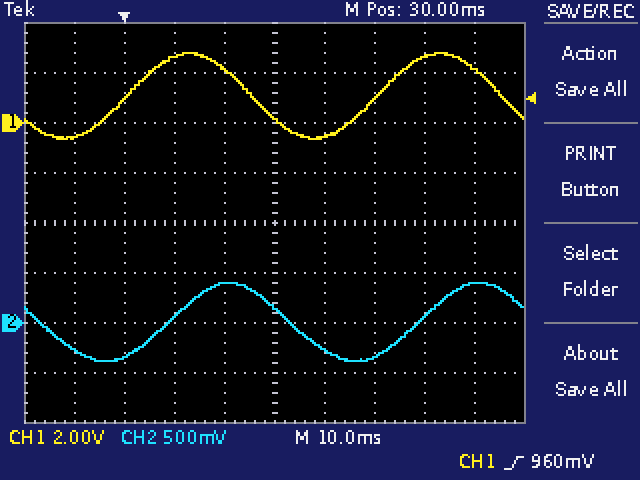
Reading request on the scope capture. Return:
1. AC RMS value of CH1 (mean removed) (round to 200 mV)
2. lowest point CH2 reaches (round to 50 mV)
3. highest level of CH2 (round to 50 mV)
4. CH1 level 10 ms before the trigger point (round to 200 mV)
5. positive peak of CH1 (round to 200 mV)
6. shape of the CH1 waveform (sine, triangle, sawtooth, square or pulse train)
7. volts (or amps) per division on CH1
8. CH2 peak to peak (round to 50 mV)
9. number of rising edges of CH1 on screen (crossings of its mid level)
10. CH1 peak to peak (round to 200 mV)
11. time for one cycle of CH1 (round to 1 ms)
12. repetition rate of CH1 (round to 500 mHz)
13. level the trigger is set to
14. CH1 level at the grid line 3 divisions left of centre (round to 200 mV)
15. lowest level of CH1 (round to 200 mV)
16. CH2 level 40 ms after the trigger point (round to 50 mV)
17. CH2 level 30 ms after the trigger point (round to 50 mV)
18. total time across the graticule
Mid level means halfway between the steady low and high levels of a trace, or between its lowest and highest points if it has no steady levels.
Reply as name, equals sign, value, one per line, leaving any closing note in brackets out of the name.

AC RMS value of CH1 (mean removed) = 1.2 V
lowest point CH2 reaches = -400 mV
highest level of CH2 = 400 mV
CH1 level 10 ms before the trigger point = -600 mV
positive peak of CH1 = 2.8 V
shape of the CH1 waveform = sine
volts (or amps) per division on CH1 = 2 V
CH2 peak to peak = 800 mV
number of rising edges of CH1 on screen = 2
CH1 peak to peak = 3.4 V
time for one cycle of CH1 = 50 ms
repetition rate of CH1 = 20.0 Hz
level the trigger is set to = 960 mV
CH1 level at the grid line 3 divisions left of centre = 1.0 V
lowest level of CH1 = -600 mV
CH2 level 40 ms after the trigger point = -250 mV
CH2 level 30 ms after the trigger point = 150 mV
total time across the graticule = 100 ms
